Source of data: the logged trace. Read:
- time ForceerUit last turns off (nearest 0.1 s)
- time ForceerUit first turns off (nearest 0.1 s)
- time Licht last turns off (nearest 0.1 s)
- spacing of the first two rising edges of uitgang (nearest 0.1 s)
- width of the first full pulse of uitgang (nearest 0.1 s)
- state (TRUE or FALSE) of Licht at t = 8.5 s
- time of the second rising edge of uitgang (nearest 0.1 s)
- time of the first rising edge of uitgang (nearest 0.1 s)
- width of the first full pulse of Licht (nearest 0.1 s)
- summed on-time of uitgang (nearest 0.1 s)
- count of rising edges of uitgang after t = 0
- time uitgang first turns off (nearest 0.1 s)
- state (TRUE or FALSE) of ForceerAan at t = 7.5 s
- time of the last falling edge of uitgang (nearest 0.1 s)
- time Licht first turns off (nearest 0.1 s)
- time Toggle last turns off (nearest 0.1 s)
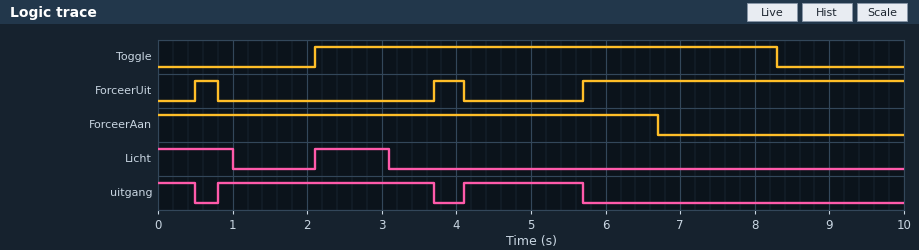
4.1 s
0.8 s
3.1 s
3.3 s
2.9 s
FALSE
4.1 s
0.8 s
1.0 s
5.0 s
2
0.5 s
FALSE
5.7 s
1.0 s
8.3 s
